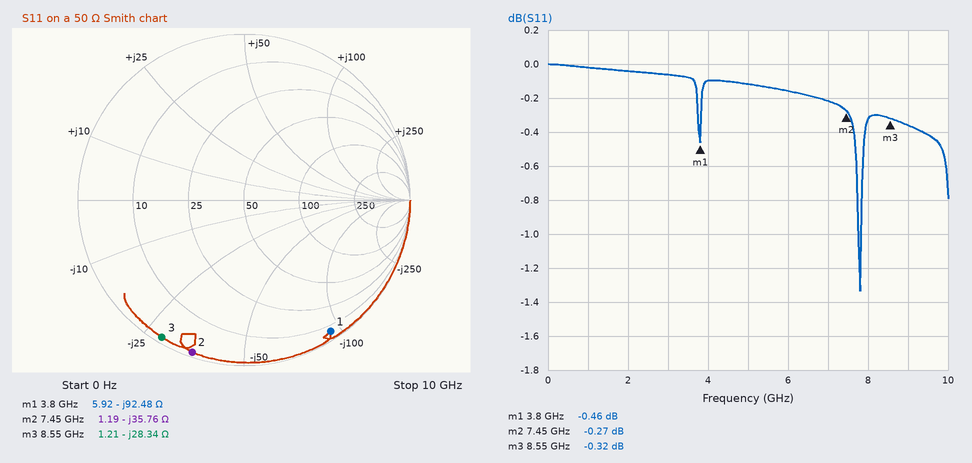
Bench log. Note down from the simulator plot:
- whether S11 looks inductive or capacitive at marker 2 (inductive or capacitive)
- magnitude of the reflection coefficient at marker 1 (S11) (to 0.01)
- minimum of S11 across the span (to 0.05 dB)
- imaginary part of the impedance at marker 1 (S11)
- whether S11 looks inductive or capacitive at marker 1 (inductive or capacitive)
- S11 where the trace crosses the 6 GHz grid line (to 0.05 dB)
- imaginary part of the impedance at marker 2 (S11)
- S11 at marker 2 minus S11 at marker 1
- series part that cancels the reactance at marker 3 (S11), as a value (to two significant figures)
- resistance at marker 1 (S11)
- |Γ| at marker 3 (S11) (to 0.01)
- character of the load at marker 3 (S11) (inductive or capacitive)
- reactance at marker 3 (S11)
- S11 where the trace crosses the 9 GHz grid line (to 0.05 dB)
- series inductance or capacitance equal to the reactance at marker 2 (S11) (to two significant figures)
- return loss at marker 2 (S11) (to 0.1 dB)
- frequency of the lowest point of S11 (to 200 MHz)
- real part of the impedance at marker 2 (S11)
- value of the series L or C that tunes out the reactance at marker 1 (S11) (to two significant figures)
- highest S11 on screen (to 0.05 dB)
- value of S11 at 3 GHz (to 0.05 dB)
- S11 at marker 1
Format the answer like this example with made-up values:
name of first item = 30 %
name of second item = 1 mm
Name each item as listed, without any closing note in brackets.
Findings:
whether S11 looks inductive or capacitive at marker 2 = capacitive
magnitude of the reflection coefficient at marker 1 (S11) = 0.95
minimum of S11 across the span = -1.35 dB
imaginary part of the impedance at marker 1 = -92.48 Ω
whether S11 looks inductive or capacitive at marker 1 = capacitive
S11 where the trace crosses the 6 GHz grid line = -0.15 dB
imaginary part of the impedance at marker 2 = -35.76 Ω
S11 at marker 2 minus S11 at marker 1 = 0.19 dB
series part that cancels the reactance at marker 3 (S11), as a value = 530 pH
resistance at marker 1 = 5.92 Ω
|Γ| at marker 3 (S11) = 0.96
character of the load at marker 3 (S11) = capacitive
reactance at marker 3 = -28.34 Ω
S11 where the trace crosses the 9 GHz grid line = -0.35 dB
series inductance or capacitance equal to the reactance at marker 2 (S11) = 600 fF
return loss at marker 2 (S11) = 0.3 dB
frequency of the lowest point of S11 = 7.8 GHz
real part of the impedance at marker 2 = 1.19 Ω
value of the series L or C that tunes out the reactance at marker 1 (S11) = 3.9 nH
highest S11 on screen = 0.00 dB
value of S11 at 3 GHz = -0.05 dB
S11 at marker 1 = -0.46 dB
